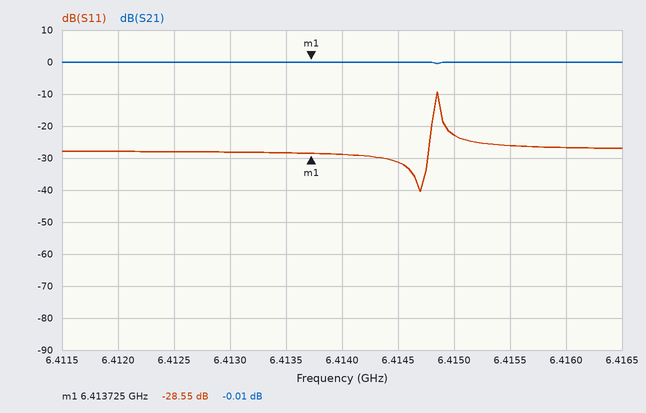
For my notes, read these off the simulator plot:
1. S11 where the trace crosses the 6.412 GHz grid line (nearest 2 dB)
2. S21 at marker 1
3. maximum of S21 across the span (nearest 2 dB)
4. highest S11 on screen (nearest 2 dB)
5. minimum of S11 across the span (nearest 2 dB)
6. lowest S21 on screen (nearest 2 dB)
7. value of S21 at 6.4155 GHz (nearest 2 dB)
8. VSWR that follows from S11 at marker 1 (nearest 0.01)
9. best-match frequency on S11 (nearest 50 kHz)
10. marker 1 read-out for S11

-28 dB
-0.01 dB
0 dB
-10 dB
-40 dB
0 dB
0 dB
1.08
6.41470 GHz
-28.55 dB
